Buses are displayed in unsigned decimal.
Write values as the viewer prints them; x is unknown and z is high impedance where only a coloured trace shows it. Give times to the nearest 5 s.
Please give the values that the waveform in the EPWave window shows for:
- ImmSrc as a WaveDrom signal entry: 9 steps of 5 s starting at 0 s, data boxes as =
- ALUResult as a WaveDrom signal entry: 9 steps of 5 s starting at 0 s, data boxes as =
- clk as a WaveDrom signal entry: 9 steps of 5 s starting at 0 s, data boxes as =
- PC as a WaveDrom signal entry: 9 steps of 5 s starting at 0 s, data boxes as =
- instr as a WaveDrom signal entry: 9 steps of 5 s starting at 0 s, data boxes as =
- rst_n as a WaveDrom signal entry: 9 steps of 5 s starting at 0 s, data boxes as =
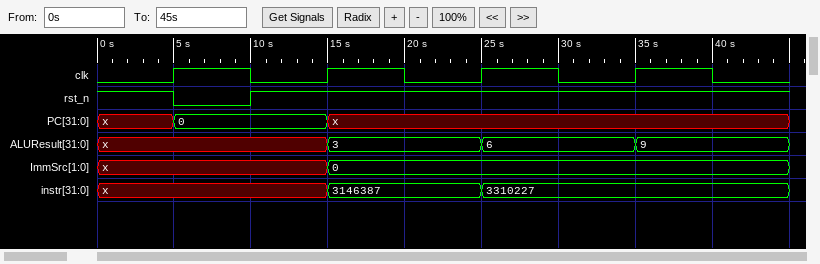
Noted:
{name: 'ImmSrc', wave: 'x..=.....', data: '0'}
{name: 'ALUResult', wave: 'x..=.=.=.', data: '3 6 9'}
{name: 'clk', wave: '010101010'}
{name: 'PC', wave: 'x=.x.....', data: '0'}
{name: 'instr', wave: 'x..=.=...', data: '3146387 3310227'}
{name: 'rst_n', wave: '101......'}
